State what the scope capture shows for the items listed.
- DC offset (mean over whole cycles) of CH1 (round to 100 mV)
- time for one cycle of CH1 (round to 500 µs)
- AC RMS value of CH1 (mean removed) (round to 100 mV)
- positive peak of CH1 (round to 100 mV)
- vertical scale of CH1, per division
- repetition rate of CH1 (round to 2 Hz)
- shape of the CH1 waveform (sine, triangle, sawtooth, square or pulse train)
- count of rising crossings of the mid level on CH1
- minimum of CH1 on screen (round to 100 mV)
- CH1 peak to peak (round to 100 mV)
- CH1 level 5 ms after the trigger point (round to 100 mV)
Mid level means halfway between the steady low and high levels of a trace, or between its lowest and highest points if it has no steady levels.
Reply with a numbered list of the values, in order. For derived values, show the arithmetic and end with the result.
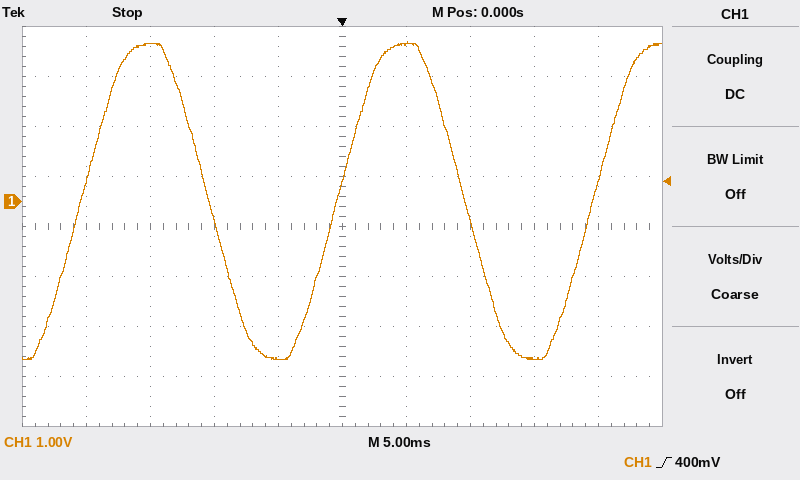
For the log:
1. (3.2 V + (-3.2 V)) / 2 ≈ 0.0 V
2. 20.0 ms
3. 6.4 V / (2√2) ≈ 2.3 V
4. 3.2 V
5. 1 V
6. 1 / 20.0 ms ≈ 50 Hz
7. sine
8. 3
9. -3.2 V
10. 3.2 V − (-3.2 V) = 6.4 V
11. 3.2 V
